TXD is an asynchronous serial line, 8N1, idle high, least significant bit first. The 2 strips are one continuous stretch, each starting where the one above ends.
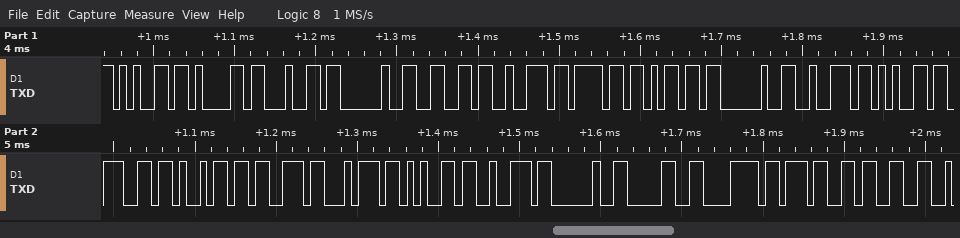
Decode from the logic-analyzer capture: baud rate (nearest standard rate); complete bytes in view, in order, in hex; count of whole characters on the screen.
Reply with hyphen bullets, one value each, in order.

- 115200 baud
- 65 61 64 20 66 72 6F 6D 20 72 65 67 69 73 74 65 72 20 30 78 37 33
- 22
